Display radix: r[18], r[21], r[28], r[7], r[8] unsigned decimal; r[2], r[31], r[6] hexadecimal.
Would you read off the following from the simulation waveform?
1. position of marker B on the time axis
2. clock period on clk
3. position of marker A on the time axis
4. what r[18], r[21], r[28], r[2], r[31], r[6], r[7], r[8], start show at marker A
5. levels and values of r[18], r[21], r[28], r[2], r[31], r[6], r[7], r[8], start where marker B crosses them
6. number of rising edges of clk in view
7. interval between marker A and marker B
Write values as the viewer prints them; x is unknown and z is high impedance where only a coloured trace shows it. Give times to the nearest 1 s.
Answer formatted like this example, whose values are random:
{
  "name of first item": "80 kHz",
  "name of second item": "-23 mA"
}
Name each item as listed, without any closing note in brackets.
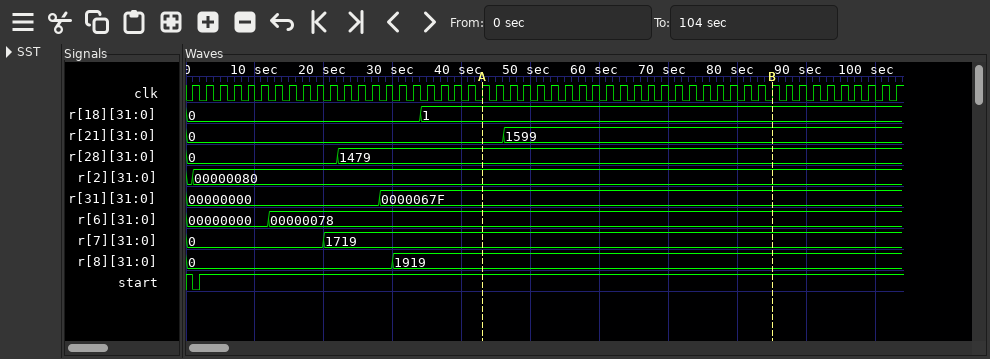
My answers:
{
  "position of marker B on the time axis": "85 s",
  "clock period on clk": "2 s",
  "position of marker A on the time axis": "43 s",
  "what r[18], r[21], r[28], r[2], r[31], r[6], r[7], r[8], start show at marker A": "r[18]=1, r[21]=0, r[28]=1479, r[2]=00000080, r[31]=0000067F, r[6]=00000078, r[7]=1719, r[8]=1919, start=1",
  "levels and values of r[18], r[21], r[28], r[2], r[31], r[6], r[7], r[8], start where marker B crosses them": "r[18]=1, r[21]=1599, r[28]=1479, r[2]=00000080, r[31]=0000067F, r[6]=00000078, r[7]=1719, r[8]=1919, start=1",
  "number of rising edges of clk in view": "52",
  "interval between marker A and marker B": "42 s"
}
